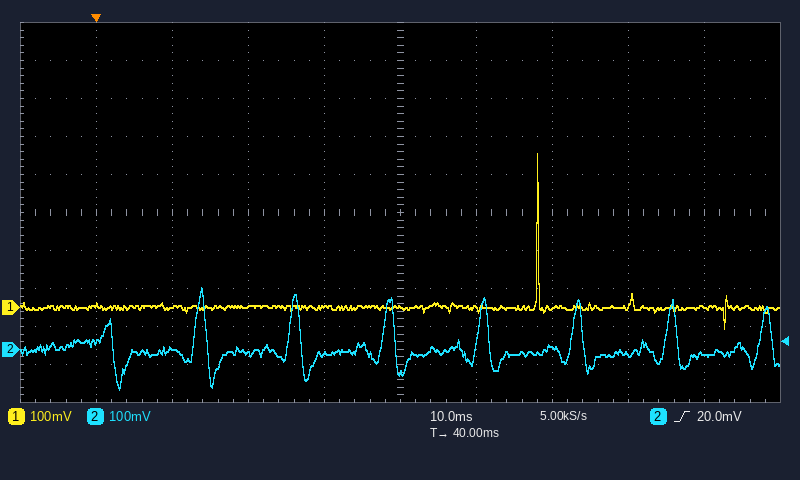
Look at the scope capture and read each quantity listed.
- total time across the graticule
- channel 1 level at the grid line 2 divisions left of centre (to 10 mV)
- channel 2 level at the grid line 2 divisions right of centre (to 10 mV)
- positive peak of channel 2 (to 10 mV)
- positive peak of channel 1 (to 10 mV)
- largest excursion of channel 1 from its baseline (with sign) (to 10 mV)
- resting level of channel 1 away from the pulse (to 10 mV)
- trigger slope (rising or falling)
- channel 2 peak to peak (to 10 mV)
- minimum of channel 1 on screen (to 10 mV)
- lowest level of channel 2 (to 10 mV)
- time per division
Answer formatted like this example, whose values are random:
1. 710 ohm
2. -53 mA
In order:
1. 100 ms
2. 0 mV
3. 10 mV
4. 160 mV
5. 410 mV
6. +410 mV
7. 0 mV
8. rising
9. 270 mV
10. -60 mV
11. -110 mV
12. 10 ms
